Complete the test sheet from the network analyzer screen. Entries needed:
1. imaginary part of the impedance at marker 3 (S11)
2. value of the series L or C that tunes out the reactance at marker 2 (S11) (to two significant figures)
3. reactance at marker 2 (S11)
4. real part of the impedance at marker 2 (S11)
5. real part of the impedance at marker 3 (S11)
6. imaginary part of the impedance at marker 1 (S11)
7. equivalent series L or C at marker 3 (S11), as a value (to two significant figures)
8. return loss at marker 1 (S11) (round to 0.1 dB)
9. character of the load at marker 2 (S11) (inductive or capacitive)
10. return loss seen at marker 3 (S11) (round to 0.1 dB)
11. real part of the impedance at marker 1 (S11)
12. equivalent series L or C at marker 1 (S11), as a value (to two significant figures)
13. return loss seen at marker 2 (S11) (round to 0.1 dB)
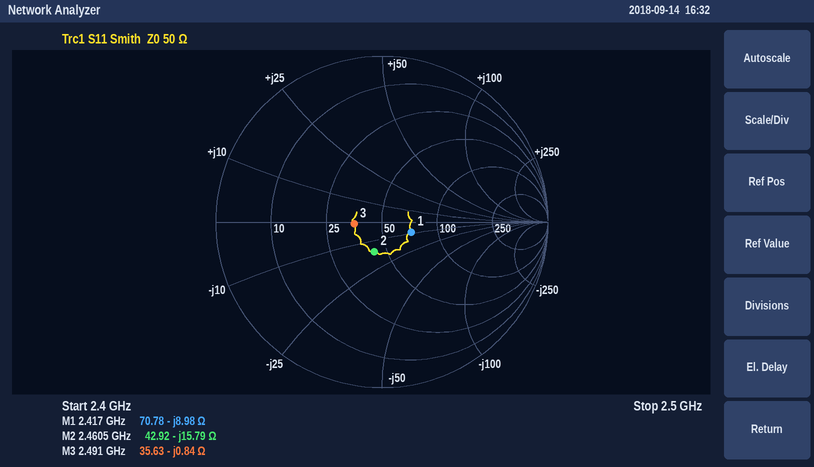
-0.84 Ω
1.0 nH
-15.79 Ω
42.92 Ω
35.63 Ω
-8.98 Ω
76 pF
14.6 dB
capacitive
15.5 dB
70.78 Ω
7.3 pF
14.7 dB
